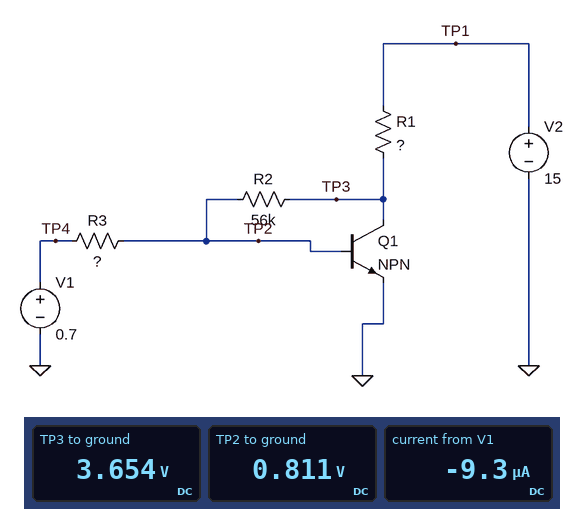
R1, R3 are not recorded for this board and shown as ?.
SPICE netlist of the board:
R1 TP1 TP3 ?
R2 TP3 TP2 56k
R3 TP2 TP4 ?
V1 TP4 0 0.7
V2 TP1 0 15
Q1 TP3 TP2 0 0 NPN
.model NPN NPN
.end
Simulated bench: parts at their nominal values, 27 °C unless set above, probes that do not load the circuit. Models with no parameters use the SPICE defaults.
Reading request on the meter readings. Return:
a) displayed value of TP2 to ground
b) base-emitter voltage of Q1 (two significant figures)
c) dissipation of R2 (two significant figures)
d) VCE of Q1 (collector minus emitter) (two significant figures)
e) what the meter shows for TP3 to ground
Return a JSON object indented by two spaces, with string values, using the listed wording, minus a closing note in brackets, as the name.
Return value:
{
  "displayed value of TP2 to ground": "0.811 V",
  "base-emitter voltage of Q1": "810 mV",
  "dissipation of R2": "140 µW",
  "VCE of Q1 (collector minus emitter)": "3.7 V",
  "what the meter shows for TP3 to ground": "3.654 V"
}
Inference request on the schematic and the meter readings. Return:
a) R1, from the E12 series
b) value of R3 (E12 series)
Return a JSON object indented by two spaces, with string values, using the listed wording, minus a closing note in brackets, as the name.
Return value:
{
  "R1, from the E12 series": "2.7 kΩ",
  "value of R3": "12 kΩ"
}
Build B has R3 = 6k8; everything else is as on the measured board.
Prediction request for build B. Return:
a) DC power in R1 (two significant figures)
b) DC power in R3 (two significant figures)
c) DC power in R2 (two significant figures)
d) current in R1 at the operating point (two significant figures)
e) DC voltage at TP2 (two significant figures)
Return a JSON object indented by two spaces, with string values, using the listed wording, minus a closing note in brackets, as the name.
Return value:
{
  "DC power in R1": "45 mW",
  "DC power in R3": "1.8 µW",
  "DC power in R2": "180 µW",
  "current in R1 at the operating point": "4.1 mA",
  "DC voltage at TP2": "810 mV"
}
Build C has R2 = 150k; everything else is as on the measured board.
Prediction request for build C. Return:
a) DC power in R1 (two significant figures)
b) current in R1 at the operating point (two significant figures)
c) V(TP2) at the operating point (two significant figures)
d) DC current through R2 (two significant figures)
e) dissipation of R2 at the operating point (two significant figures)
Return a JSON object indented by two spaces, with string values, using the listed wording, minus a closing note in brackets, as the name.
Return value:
{
  "DC power in R1": "26 mW",
  "current in R1 at the operating point": "3.1 mA",
  "V(TP2) at the operating point": "800 mV",
  "DC current through R2": "39 µA",
  "dissipation of R2 at the operating point": "230 µW"
}
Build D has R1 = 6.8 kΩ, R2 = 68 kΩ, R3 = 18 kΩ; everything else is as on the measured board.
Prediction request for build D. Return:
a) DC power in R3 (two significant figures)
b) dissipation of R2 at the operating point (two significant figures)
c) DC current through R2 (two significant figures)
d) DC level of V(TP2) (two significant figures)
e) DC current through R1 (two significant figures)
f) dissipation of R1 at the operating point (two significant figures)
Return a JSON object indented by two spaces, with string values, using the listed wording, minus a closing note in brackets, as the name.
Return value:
{
  "DC power in R3": "450 nW",
  "dissipation of R2 at the operating point": "37 µW",
  "DC current through R2": "23 µA",
  "DC level of V(TP2)": "790 mV",
  "DC current through R1": "1.9 mA",
  "dissipation of R1 at the operating point": "23 mW"
}
